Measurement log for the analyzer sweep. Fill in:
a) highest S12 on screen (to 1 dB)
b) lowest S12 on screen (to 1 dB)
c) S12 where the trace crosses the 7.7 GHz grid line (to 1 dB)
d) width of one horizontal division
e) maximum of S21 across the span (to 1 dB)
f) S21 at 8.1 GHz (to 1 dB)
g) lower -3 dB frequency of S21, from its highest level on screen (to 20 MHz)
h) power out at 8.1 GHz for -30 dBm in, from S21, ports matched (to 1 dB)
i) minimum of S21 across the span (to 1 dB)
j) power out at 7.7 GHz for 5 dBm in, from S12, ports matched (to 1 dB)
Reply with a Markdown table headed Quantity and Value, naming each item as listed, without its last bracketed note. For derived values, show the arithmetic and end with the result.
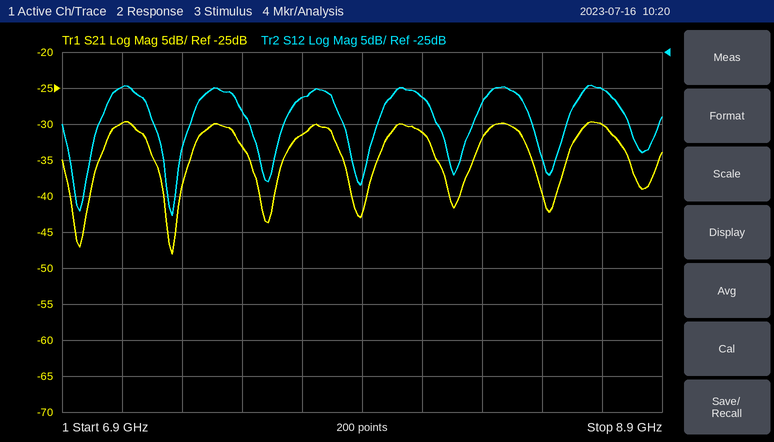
| Quantity | Value |
|---|---|
| highest S12 on screen | -30 dB |
| lowest S12 on screen | -48 dB |
| S12 where the trace crosses the 7.7 GHz grid line | -31 dB |
| width of one horizontal division | 200 MHz |
| maximum of S21 across the span | -30 dB |
| S21 at 8.1 GHz | -31 dB |
| lower -3 dB frequency of S21, from its highest level on screen | 7.04 GHz |
| power out at 8.1 GHz for -30 dBm in, from S21, ports matched | -30 dBm + (-31 dB) = -61 dBm |
| minimum of S21 across the span | -48 dB |
| power out at 7.7 GHz for 5 dBm in, from S12, ports matched | 5 dBm + (-31 dB) = -26 dBm |
